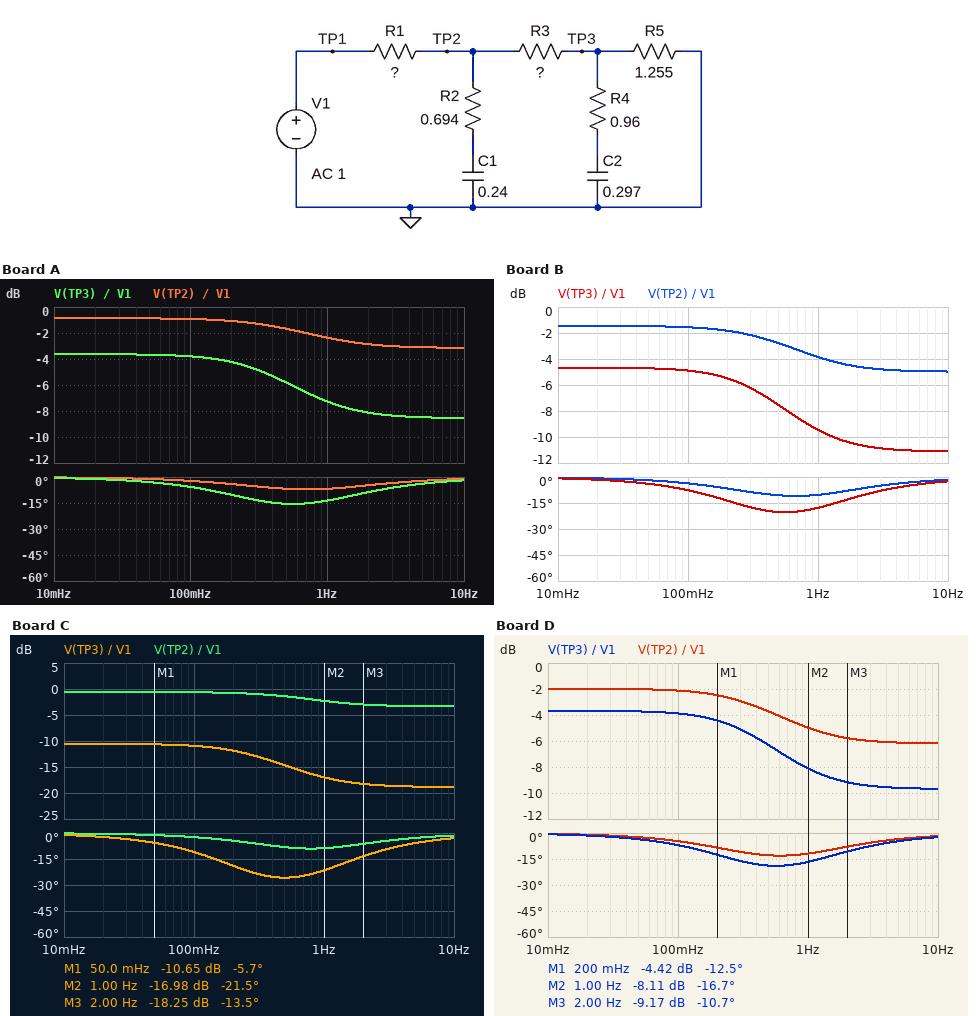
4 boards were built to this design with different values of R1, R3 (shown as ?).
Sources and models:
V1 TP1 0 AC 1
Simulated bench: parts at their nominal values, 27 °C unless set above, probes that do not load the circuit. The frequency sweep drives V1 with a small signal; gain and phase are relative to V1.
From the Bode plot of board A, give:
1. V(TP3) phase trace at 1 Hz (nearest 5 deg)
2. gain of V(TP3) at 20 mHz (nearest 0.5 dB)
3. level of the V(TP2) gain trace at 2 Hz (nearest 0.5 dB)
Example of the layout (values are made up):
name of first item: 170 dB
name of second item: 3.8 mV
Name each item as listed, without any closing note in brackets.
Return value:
V(TP3) phase trace at 1 Hz: -15 deg
gain of V(TP3) at 20 mHz: -3.5 dB
level of the V(TP2) gain trace at 2 Hz: -3.0 dB
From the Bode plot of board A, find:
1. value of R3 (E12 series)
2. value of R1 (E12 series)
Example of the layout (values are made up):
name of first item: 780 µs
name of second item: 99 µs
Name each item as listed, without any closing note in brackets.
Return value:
value of R3: 0.47 Ω
value of R1: 0.18 Ω
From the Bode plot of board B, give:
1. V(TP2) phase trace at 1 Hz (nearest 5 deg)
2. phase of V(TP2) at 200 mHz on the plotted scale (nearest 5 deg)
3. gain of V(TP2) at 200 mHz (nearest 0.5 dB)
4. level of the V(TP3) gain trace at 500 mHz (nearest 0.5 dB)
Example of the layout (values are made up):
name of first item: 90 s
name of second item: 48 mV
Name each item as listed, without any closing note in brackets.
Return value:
V(TP2) phase trace at 1 Hz: -10 deg
phase of V(TP2) at 200 mHz on the plotted scale: -5 deg
gain of V(TP2) at 200 mHz: -2.0 dB
level of the V(TP3) gain trace at 500 mHz: -7.5 dB
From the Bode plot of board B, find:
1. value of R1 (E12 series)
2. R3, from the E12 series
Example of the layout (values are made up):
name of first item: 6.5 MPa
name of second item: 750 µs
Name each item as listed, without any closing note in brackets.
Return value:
value of R1: 0.33 Ω
R3, from the E12 series: 0.56 Ω
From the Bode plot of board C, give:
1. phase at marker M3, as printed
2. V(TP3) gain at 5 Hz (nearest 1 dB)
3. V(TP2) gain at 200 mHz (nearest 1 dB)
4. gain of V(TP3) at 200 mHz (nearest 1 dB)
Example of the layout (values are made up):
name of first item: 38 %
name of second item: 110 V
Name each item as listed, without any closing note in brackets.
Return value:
phase at marker M3, as printed: -13.5 deg
V(TP3) gain at 5 Hz: -19 dB
V(TP2) gain at 200 mHz: -1 dB
gain of V(TP3) at 200 mHz: -12 dB
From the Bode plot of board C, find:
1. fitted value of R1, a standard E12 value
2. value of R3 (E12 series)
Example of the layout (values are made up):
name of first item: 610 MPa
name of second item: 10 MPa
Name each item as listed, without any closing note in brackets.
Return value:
fitted value of R1, a standard E12 value: 0.27 Ω
value of R3: 2.7 Ω
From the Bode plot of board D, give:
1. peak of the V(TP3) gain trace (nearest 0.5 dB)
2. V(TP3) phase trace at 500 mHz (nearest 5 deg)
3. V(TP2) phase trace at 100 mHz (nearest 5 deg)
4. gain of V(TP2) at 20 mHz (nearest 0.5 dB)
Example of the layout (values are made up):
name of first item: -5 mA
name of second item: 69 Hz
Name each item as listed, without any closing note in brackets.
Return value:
peak of the V(TP3) gain trace: -3.5 dB
V(TP3) phase trace at 500 mHz: -20 deg
V(TP2) phase trace at 100 mHz: -5 deg
gain of V(TP2) at 20 mHz: -2.0 dB
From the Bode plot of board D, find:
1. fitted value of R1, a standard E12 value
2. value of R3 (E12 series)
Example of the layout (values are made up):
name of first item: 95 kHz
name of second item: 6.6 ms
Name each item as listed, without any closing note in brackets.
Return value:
fitted value of R1, a standard E12 value: 0.39 Ω
value of R3: 0.27 Ω
